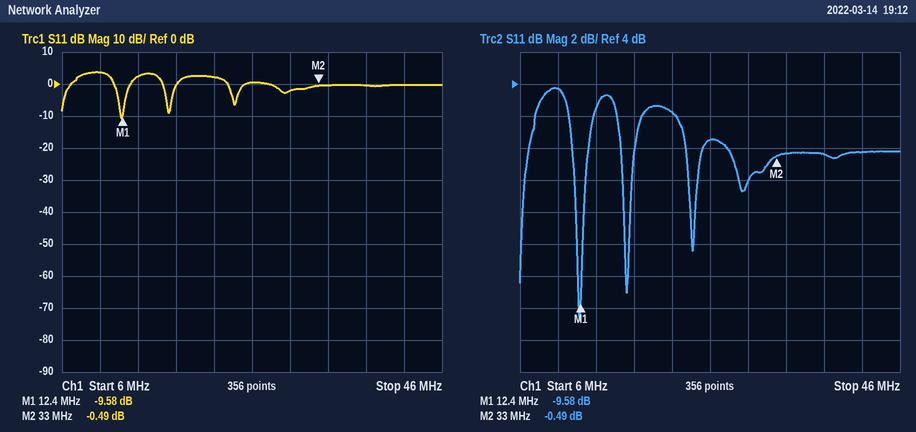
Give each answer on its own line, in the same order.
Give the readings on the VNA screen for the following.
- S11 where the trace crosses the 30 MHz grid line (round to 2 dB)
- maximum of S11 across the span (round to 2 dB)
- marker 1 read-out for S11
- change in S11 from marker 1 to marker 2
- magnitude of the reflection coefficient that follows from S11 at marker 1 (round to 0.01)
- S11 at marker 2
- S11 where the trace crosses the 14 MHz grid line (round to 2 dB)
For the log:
-2 dB
4 dB
-9.58 dB
9.09 dB
0.33
-0.49 dB
2 dB
